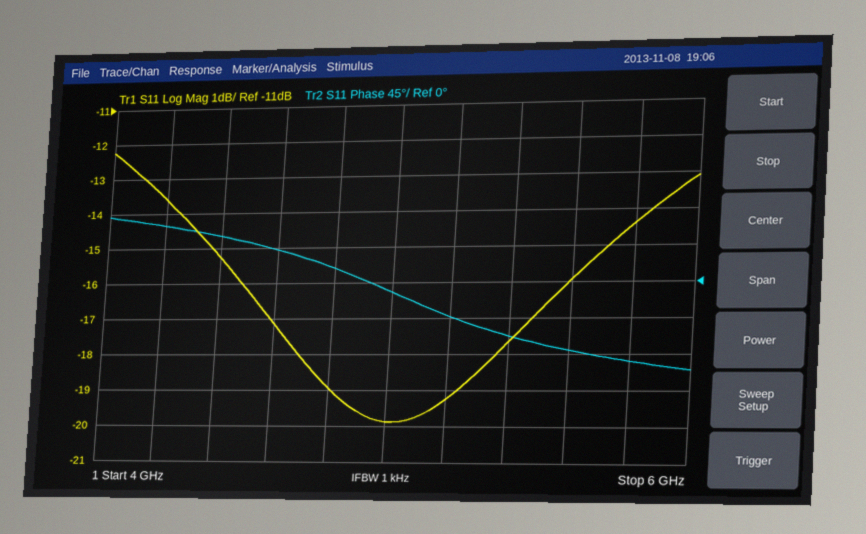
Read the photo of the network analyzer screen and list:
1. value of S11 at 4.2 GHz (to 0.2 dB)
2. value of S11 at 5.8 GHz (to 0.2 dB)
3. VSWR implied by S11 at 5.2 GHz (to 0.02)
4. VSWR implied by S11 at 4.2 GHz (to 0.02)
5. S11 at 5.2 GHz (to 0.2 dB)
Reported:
-13.6 dB
-14.4 dB
1.24
1.52
-19.2 dB
